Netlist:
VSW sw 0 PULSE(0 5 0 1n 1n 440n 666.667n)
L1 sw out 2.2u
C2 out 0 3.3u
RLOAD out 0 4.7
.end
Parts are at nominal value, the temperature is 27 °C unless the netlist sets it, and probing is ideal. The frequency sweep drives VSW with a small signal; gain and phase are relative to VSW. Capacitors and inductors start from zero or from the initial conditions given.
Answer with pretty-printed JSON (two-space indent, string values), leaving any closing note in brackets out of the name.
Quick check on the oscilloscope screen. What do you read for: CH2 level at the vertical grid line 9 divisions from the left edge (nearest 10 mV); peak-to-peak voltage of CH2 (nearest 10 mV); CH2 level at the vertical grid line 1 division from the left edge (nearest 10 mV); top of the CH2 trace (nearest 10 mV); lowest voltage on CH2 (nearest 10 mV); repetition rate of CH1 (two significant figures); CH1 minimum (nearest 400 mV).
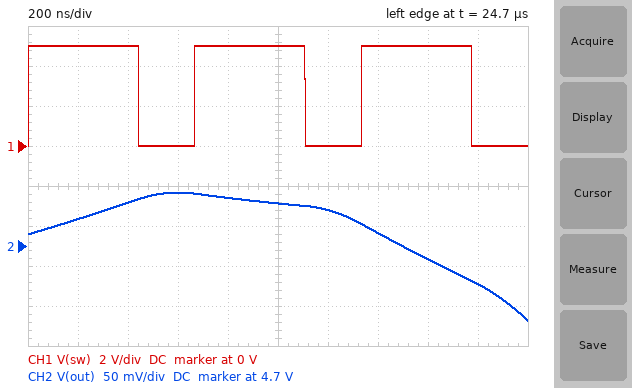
{
  "CH2 level at the vertical grid line 9 divisions from the left edge": "4.65 V",
  "peak-to-peak voltage of CH2": "160 mV",
  "CH2 level at the vertical grid line 1 division from the left edge": "4.73 V",
  "top of the CH2 trace": "4.77 V",
  "lowest voltage on CH2": "4.61 V",
  "repetition rate of CH1": "1.5 MHz",
  "CH1 minimum": "0 V"
}
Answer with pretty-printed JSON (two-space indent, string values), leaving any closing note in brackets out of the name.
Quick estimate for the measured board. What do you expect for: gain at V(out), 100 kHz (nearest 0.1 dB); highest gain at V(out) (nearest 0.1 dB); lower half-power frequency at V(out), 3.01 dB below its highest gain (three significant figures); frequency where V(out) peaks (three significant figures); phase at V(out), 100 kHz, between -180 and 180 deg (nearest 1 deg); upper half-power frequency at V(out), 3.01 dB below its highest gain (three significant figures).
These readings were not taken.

{
  "gain at V(out), 100 kHz": "-5.5 dB",
  "highest gain at V(out)": "15.2 dB",
  "lower half-power frequency at V(out), 3.01 dB below its highest gain": "53.2 kHz",
  "frequency where V(out) peaks": "58.6 kHz",
  "phase at V(out), 100 kHz, between -180 and 180 deg": "-171 deg",
  "upper half-power frequency at V(out), 3.01 dB below its highest gain": "63.6 kHz"
}
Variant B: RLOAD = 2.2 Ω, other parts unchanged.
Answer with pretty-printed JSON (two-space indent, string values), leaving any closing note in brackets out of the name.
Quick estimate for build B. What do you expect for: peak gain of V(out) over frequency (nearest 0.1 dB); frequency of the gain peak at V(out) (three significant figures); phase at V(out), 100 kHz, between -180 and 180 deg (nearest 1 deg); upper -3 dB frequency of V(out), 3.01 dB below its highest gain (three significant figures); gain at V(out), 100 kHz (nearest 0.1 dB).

{
  "peak gain of V(out) over frequency": "8.8 dB",
  "frequency of the gain peak at V(out)": "57.0 kHz",
  "phase at V(out), 100 kHz, between -180 and 180 deg": "-161 deg",
  "upper -3 dB frequency of V(out), 3.01 dB below its highest gain": "67.2 kHz",
  "gain at V(out), 100 kHz": "-5.9 dB"
}
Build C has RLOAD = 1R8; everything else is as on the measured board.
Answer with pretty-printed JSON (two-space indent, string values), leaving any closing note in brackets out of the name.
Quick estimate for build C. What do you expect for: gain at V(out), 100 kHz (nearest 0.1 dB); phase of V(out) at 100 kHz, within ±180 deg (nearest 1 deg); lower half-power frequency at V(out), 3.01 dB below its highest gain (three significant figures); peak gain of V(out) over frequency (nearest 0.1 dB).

{
  "gain at V(out), 100 kHz": "-6.1 dB",
  "phase of V(out) at 100 kHz, within ±180 deg": "-158 deg",
  "lower half-power frequency at V(out), 3.01 dB below its highest gain": "39.9 kHz",
  "peak gain of V(out) over frequency": "7.1 dB"
}
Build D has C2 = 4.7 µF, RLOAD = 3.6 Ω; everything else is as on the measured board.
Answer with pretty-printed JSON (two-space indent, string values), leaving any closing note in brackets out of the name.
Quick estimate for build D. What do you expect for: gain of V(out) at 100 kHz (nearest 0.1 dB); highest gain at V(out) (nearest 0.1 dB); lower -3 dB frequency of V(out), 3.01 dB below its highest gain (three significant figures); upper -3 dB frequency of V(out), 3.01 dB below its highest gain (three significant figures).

{
  "gain of V(out) at 100 kHz": "-9.8 dB",
  "highest gain at V(out)": "14.5 dB",
  "lower -3 dB frequency of V(out), 3.01 dB below its highest gain": "44.1 kHz",
  "upper -3 dB frequency of V(out), 3.01 dB below its highest gain": "53.6 kHz"
}
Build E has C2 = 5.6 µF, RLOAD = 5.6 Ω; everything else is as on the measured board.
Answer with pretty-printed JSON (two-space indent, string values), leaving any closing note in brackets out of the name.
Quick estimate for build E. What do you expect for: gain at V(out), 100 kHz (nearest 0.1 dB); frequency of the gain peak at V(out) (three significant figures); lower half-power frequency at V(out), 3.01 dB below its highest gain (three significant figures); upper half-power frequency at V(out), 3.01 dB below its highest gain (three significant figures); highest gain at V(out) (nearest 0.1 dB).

{
  "gain at V(out), 100 kHz": "-11.8 dB",
  "frequency of the gain peak at V(out)": "45.2 kHz",
  "lower half-power frequency at V(out), 3.01 dB below its highest gain": "42.6 kHz",
  "upper half-power frequency at V(out), 3.01 dB below its highest gain": "47.7 kHz",
  "highest gain at V(out)": "19.0 dB"
}
